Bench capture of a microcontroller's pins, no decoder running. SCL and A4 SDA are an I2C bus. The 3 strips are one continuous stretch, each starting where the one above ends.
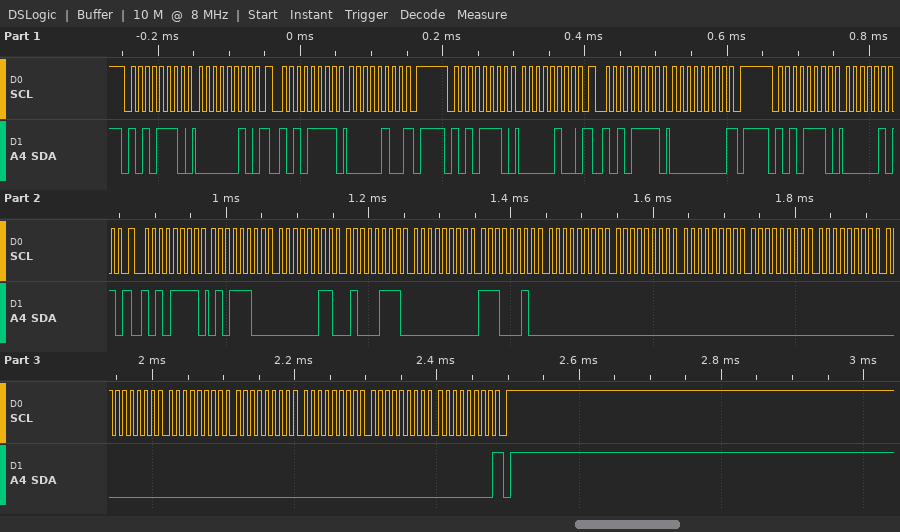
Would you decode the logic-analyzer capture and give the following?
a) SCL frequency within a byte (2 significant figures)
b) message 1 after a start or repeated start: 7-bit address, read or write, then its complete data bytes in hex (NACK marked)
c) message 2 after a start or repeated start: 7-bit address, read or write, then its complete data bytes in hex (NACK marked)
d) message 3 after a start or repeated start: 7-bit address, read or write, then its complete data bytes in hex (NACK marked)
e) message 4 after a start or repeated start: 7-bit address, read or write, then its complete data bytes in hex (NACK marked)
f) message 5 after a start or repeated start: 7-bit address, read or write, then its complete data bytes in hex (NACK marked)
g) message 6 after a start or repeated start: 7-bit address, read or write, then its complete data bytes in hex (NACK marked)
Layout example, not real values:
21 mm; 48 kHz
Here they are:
100 kHz; 0x57 write: 02; 0x57 read: 04 NACK; 0x57 write: 04; 0x57 read: 00 NACK; 0x57 write: 05; 0x57 read: 5C 03 47 00 E2 00 00 00 00 00 00 00 00 00 00 00 NACK
